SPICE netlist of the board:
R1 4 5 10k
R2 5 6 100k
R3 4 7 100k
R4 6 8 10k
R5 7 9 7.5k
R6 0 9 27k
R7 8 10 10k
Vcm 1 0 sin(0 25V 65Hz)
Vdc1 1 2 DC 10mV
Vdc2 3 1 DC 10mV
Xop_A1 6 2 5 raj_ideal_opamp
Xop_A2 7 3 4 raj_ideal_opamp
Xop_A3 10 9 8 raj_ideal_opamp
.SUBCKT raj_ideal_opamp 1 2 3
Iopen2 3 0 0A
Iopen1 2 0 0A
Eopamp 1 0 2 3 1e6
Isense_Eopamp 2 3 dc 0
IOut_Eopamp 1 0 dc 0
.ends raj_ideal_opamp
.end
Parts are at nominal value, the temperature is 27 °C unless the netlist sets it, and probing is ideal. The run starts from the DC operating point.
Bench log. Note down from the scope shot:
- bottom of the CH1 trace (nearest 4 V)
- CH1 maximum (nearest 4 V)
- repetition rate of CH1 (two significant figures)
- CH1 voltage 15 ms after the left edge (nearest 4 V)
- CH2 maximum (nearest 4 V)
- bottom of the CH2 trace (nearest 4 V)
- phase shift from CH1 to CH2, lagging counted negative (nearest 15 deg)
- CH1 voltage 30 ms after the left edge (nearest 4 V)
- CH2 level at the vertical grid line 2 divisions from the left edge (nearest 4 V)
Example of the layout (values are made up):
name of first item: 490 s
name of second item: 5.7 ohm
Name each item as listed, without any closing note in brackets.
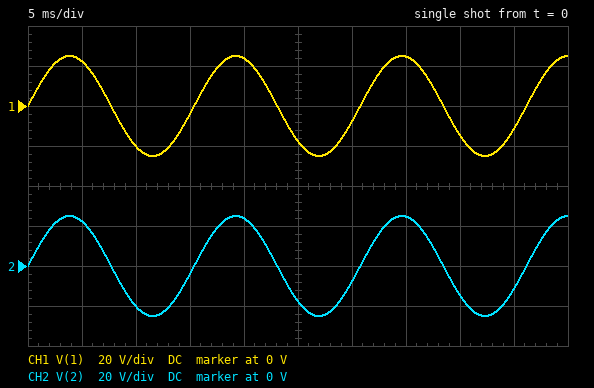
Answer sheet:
bottom of the CH1 trace: -24 V
CH1 maximum: 24 V
repetition rate of CH1: 65 Hz
CH1 voltage 15 ms after the left edge: -4 V
CH2 maximum: 24 V
bottom of the CH2 trace: -24 V
phase shift from CH1 to CH2, lagging counted negative: 0 deg
CH1 voltage 30 ms after the left edge: -8 V
CH2 level at the vertical grid line 2 divisions from the left edge: -20 V
